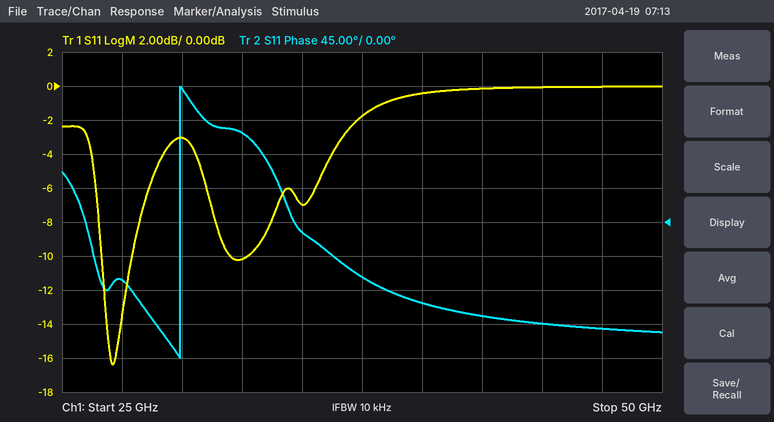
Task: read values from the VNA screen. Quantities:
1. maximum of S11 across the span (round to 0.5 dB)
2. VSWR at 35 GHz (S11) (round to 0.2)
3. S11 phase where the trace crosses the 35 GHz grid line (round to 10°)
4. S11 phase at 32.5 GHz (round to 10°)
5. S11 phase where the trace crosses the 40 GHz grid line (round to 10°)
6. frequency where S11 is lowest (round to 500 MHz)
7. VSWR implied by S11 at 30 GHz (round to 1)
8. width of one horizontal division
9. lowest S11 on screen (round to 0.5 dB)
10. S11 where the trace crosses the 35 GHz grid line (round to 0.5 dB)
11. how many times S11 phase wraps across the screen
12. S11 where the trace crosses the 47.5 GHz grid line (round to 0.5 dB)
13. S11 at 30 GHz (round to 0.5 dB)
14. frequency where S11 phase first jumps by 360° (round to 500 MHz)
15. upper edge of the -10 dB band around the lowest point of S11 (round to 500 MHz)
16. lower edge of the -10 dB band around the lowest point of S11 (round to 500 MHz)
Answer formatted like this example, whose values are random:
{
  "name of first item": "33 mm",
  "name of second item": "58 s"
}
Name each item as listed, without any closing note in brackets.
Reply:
{
  "maximum of S11 across the span": "0.0 dB",
  "VSWR at 35 GHz (S11)": "2.6",
  "S11 phase where the trace crosses the 35 GHz grid line": "-10°",
  "S11 phase at 32.5 GHz": "120°",
  "S11 phase where the trace crosses the 40 GHz grid line": "-110°",
  "frequency where S11 is lowest": "27.0 GHz",
  "VSWR implied by S11 at 30 GHz": "6",
  "width of one horizontal division": "2.5 GHz",
  "lowest S11 on screen": "-16.5 dB",
  "S11 where the trace crosses the 35 GHz grid line": "-7.0 dB",
  "how many times S11 phase wraps across the screen": "1",
  "S11 where the trace crosses the 47.5 GHz grid line": "0.0 dB",
  "S11 at 30 GHz": "-3.0 dB",
  "frequency where S11 phase first jumps by 360°": "30.0 GHz",
  "upper edge of the -10 dB band around the lowest point of S11": "28.0 GHz",
  "lower edge of the -10 dB band around the lowest point of S11": "26.5 GHz"
}
